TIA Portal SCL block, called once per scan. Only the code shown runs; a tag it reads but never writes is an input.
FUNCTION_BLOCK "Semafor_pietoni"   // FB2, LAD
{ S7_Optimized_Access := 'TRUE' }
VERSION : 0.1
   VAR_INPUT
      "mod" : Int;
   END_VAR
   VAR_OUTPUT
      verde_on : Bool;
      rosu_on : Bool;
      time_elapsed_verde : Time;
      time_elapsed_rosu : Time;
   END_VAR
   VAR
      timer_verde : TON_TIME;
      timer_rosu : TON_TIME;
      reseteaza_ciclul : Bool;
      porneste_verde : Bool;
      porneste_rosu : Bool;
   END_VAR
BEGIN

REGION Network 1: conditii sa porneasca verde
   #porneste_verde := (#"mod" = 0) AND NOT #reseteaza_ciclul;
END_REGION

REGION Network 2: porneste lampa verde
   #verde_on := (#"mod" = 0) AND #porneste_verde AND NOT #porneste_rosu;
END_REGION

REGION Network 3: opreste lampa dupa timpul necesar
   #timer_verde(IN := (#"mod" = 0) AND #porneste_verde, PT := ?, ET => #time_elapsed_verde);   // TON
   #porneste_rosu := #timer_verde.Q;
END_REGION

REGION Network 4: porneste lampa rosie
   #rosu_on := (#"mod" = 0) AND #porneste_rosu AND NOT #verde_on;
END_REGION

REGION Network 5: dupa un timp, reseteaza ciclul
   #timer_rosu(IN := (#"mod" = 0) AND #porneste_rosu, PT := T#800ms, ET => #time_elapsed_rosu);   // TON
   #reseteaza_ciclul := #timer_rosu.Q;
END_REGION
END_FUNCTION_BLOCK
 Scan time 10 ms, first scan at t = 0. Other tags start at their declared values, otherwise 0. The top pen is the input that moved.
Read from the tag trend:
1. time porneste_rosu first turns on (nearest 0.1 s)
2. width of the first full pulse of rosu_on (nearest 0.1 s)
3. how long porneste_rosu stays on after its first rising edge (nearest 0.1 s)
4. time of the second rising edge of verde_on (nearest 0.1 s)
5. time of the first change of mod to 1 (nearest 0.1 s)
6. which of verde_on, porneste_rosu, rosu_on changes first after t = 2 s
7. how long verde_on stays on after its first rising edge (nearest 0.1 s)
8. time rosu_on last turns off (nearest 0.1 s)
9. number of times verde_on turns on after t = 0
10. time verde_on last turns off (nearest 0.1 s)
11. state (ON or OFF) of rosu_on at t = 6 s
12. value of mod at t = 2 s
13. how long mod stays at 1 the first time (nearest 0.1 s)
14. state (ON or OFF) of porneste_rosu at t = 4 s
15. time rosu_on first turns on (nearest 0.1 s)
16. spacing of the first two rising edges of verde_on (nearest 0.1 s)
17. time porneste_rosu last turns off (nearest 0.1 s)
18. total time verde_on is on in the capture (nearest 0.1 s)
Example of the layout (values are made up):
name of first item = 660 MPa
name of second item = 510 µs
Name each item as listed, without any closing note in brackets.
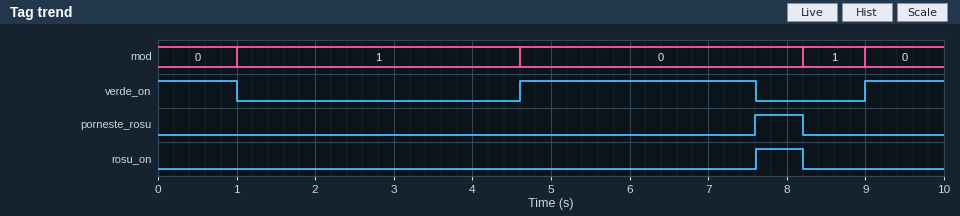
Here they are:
time porneste_rosu first turns on = 7.6 s
width of the first full pulse of rosu_on = 0.6 s
how long porneste_rosu stays on after its first rising edge = 0.6 s
time of the second rising edge of verde_on = 9.0 s
time of the first change of mod to 1 = 1.0 s
which of verde_on, porneste_rosu, rosu_on changes first after t = 2 s = verde_on
how long verde_on stays on after its first rising edge = 3.0 s
time rosu_on last turns off = 8.2 s
number of times verde_on turns on after t = 0 = 2
time verde_on last turns off = 7.6 s
state (ON or OFF) of rosu_on at t = 6 s = OFF
value of mod at t = 2 s = 1
how long mod stays at 1 the first time = 3.6 s
state (ON or OFF) of porneste_rosu at t = 4 s = OFF
time rosu_on first turns on = 7.6 s
spacing of the first two rising edges of verde_on = 4.4 s
time porneste_rosu last turns off = 8.2 s
total time verde_on is on in the capture = 5.0 s
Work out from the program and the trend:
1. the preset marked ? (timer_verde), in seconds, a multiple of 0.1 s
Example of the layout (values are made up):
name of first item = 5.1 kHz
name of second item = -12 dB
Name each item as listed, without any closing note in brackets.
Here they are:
the preset marked ? (timer_verde), in seconds, a multiple of 0.1 s = 3.0 s
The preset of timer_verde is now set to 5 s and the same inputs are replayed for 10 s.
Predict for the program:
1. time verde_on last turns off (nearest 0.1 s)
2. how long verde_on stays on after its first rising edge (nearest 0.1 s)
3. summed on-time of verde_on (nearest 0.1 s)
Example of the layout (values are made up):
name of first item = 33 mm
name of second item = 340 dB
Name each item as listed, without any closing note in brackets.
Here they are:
time verde_on last turns off = 8.2 s
how long verde_on stays on after its first rising edge = 3.6 s
summed on-time of verde_on = 5.6 s
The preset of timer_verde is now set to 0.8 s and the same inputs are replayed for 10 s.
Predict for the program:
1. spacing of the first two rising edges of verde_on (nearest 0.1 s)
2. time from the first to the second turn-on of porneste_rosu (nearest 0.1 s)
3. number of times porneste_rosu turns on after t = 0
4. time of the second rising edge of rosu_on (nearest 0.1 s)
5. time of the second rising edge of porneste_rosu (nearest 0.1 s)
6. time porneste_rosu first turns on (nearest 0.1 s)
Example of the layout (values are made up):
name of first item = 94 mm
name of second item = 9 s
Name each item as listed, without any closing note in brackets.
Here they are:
spacing of the first two rising edges of verde_on = 1.6 s
time from the first to the second turn-on of porneste_rosu = 4.6 s
number of times porneste_rosu turns on after t = 0 = 4
time of the second rising edge of rosu_on = 5.4 s
time of the second rising edge of porneste_rosu = 5.4 s
time porneste_rosu first turns on = 0.8 s
